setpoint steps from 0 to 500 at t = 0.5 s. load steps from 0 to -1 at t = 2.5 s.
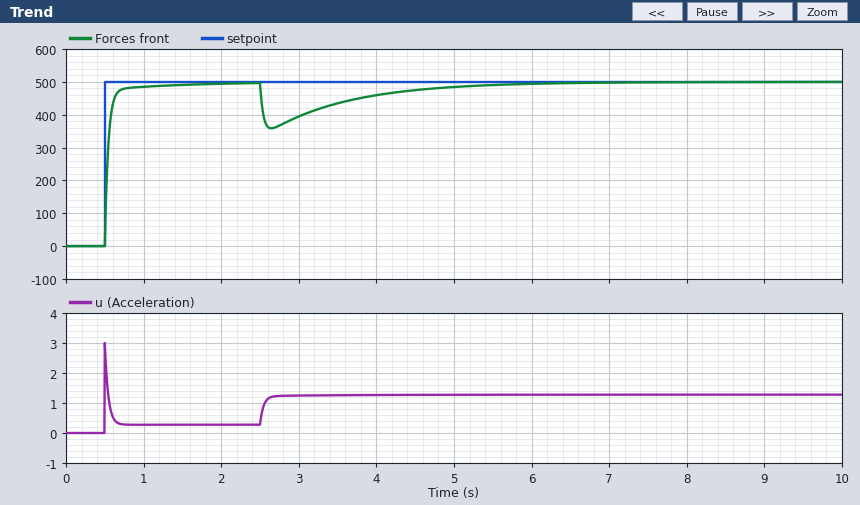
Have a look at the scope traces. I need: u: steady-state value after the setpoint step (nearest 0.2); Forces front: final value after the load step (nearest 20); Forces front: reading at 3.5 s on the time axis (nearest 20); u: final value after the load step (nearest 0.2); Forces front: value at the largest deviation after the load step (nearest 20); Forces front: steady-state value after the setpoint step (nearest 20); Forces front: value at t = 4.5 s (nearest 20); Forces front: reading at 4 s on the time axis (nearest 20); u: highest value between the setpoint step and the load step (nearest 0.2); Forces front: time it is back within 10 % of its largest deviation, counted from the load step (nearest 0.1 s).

0.2
500
440
1.2
360
500
480
460
3.0
2.6 s
